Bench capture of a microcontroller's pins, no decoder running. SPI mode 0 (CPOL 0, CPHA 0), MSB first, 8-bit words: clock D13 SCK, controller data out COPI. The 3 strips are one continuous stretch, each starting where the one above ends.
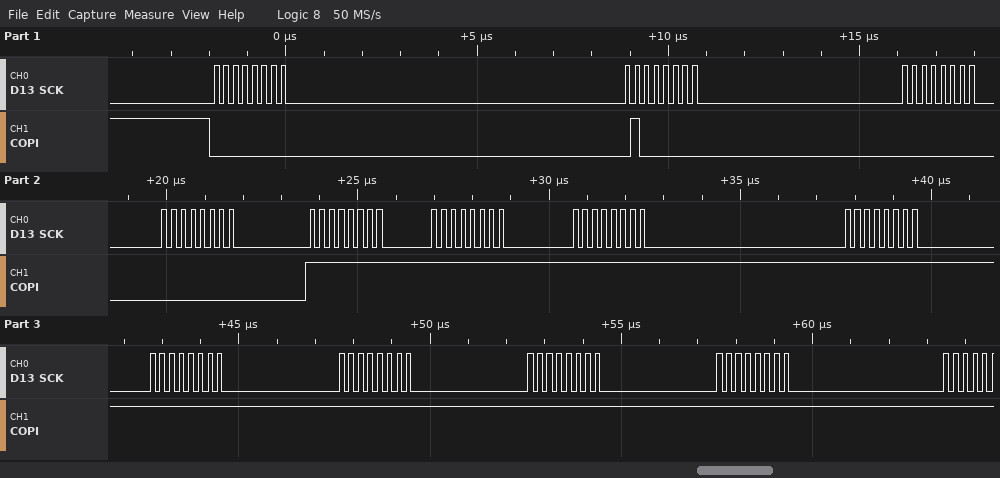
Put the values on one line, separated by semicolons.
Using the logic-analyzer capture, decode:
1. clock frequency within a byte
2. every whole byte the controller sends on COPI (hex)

4 MHz; 0x00 0x40 0x00 0x00 0xFF 0xFF 0xFF 0xFF 0xFF 0xFF 0xFF 0xFF
